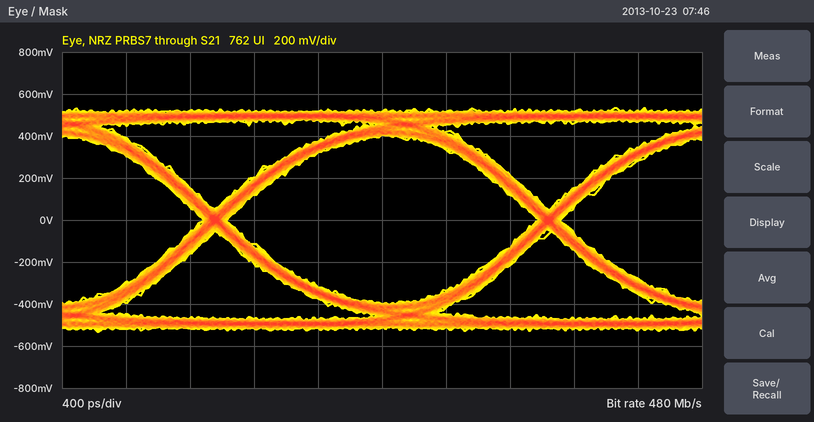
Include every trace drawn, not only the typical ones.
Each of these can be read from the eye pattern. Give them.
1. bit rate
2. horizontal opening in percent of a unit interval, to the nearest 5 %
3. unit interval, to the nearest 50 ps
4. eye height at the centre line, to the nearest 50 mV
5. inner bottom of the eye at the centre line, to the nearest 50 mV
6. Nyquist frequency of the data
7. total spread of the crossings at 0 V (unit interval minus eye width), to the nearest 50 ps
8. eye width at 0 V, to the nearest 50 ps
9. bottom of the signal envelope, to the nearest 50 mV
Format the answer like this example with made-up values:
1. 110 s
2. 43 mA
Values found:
1. 480 Mb/s
2. 95 %
3. 2.10 ns
4. 800 mV
5. -400 mV
6. 240 MHz
7. 150 ps
8. 1.95 ns
9. -550 mV
